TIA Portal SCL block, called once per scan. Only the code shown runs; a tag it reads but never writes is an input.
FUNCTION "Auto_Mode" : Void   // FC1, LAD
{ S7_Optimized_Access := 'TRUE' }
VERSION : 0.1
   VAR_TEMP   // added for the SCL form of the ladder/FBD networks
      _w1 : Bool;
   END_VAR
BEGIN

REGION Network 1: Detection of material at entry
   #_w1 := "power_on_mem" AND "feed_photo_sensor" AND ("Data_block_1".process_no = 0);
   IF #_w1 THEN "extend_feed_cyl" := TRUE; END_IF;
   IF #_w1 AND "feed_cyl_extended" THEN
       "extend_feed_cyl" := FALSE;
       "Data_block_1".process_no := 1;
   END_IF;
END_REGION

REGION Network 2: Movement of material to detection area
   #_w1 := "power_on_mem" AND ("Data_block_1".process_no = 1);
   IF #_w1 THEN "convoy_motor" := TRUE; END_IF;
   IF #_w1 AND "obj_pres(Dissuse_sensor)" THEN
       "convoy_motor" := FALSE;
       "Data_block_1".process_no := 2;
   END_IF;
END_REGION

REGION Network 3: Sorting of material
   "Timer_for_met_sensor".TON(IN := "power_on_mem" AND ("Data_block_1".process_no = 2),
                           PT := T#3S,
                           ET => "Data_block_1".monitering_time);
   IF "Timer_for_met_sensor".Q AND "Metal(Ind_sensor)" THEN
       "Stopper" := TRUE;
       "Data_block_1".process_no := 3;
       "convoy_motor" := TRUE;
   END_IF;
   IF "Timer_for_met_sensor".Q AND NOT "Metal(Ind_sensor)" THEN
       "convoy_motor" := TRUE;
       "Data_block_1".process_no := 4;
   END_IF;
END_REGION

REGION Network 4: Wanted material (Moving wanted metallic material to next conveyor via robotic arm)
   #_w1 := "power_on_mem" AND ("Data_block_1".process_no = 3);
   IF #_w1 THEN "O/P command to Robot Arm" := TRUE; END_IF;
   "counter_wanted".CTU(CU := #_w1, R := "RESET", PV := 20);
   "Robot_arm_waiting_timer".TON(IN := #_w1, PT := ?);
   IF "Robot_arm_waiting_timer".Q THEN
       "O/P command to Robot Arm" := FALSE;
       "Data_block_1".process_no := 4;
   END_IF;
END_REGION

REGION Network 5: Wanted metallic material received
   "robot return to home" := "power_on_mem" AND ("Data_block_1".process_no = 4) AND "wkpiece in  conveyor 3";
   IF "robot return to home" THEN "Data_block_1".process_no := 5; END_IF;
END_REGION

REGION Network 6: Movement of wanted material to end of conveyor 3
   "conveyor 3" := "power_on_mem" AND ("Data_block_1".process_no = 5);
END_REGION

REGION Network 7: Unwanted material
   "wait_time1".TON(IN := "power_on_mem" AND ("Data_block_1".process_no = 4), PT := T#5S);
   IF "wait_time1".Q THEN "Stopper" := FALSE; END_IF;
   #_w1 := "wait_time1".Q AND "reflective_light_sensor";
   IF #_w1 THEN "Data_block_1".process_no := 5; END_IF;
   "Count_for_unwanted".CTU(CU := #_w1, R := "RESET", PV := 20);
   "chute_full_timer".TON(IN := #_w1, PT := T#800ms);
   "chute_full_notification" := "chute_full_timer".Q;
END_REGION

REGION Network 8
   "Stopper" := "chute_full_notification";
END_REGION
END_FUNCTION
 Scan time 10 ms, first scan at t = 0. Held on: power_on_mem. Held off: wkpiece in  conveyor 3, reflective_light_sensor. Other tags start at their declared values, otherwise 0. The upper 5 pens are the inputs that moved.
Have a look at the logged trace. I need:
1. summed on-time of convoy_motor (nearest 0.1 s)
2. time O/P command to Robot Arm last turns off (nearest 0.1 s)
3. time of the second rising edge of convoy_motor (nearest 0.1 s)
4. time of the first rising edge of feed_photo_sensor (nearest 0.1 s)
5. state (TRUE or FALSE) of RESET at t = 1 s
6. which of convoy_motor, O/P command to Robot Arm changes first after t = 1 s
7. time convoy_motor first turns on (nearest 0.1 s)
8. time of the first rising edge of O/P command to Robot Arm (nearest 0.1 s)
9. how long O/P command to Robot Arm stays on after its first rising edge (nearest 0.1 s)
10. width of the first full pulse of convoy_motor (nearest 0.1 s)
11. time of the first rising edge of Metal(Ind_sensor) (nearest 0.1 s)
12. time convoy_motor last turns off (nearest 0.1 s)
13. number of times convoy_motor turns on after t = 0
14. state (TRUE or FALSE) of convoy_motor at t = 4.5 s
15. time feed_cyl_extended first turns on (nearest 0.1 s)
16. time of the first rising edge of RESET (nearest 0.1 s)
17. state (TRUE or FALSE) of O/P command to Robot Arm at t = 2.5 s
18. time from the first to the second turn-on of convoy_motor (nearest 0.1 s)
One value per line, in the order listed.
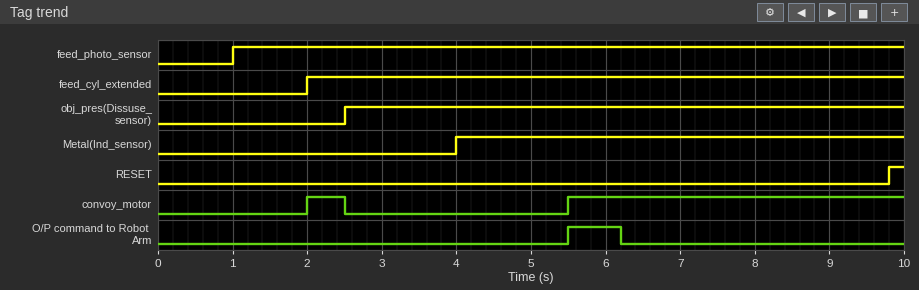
5.0 s
6.2 s
5.5 s
1.0 s
FALSE
convoy_motor
2.0 s
5.5 s
0.7 s
0.5 s
4.0 s
2.5 s
2
FALSE
2.0 s
9.8 s
FALSE
3.5 s
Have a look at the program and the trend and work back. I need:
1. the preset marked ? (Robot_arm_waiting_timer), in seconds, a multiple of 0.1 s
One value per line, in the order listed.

0.7 s
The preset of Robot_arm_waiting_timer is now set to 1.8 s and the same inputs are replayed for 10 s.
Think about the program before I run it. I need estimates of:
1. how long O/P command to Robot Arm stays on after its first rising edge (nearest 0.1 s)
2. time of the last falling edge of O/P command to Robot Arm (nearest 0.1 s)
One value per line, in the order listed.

1.8 s
7.3 s
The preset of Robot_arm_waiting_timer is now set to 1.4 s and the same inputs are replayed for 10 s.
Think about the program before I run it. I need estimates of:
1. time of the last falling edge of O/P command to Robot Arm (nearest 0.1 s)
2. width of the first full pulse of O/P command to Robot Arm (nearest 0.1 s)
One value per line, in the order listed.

6.9 s
1.4 s
